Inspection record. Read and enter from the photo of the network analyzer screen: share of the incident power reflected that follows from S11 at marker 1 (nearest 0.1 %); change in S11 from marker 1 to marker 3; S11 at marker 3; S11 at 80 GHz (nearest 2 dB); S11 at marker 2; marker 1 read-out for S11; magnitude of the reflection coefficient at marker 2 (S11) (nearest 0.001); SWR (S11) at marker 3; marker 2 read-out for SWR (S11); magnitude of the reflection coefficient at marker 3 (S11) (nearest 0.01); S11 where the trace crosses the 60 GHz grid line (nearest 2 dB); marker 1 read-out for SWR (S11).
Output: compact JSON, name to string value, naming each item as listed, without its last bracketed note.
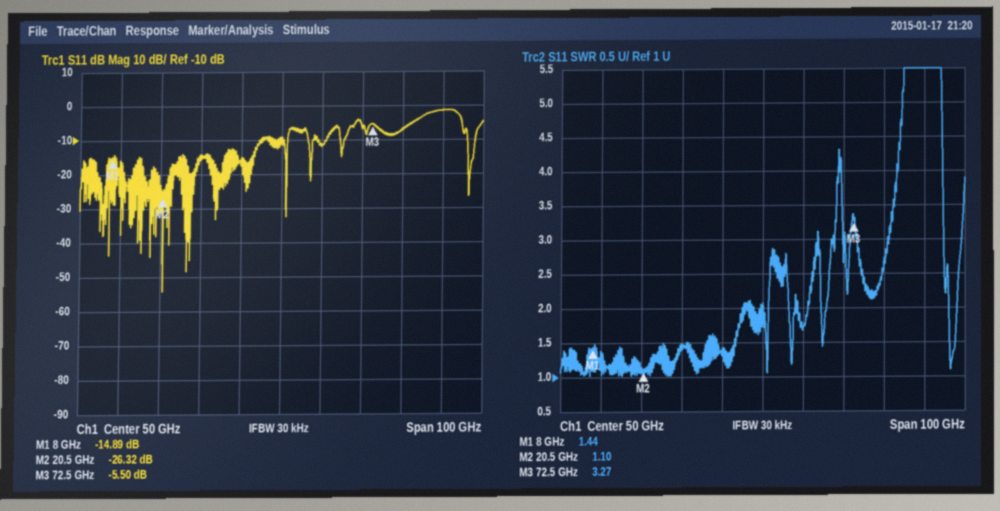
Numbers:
{"share of the incident power reflected that follows from S11 at marker 1": "3.2 %", "change in S11 from marker 1 to marker 3": "9.39 dB", "S11 at marker 3": "-5.50 dB", "S11 at 80 GHz": "-6 dB", "S11 at marker 2": "-26.32 dB", "marker 1 read-out for S11": "-14.89 dB", "magnitude of the reflection coefficient at marker 2 (S11)": "0.048", "SWR (S11) at marker 3": "3.27", "marker 2 read-out for SWR": "1.10", "magnitude of the reflection coefficient at marker 3 (S11)": "0.53", "S11 where the trace crosses the 60 GHz grid line": "-12 dB", "marker 1 read-out for SWR": "1.44"}
